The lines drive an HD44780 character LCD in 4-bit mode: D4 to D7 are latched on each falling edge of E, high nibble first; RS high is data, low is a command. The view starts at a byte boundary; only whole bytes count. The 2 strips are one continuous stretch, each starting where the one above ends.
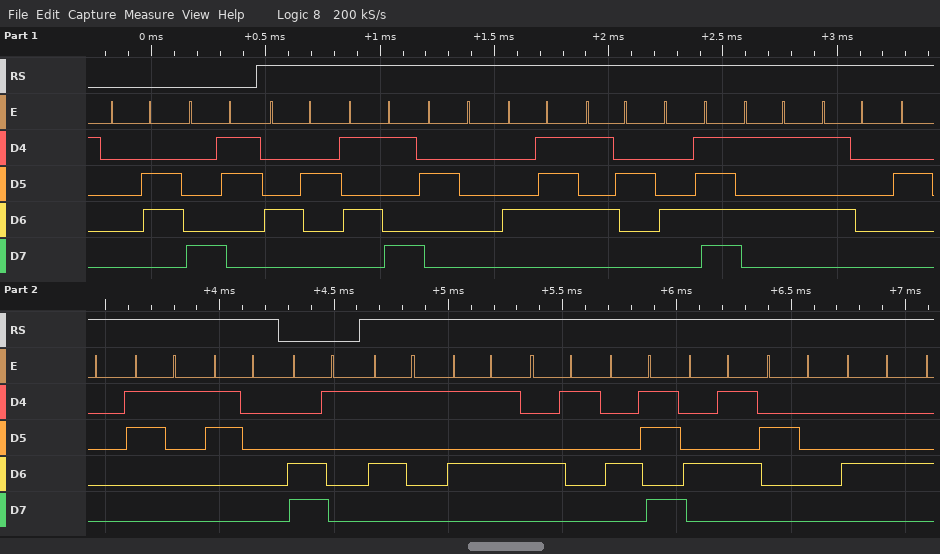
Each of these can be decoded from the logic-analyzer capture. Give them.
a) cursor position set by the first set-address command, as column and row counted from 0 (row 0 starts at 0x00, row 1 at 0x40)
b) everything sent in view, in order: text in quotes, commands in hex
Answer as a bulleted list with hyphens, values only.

- column 3, row 0
- 0x06 0x83 "BY GROUP 10" 0xC1 "QUAKE D"
